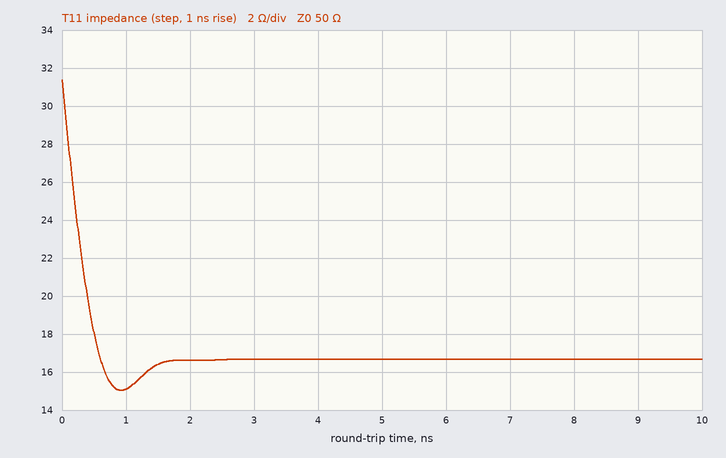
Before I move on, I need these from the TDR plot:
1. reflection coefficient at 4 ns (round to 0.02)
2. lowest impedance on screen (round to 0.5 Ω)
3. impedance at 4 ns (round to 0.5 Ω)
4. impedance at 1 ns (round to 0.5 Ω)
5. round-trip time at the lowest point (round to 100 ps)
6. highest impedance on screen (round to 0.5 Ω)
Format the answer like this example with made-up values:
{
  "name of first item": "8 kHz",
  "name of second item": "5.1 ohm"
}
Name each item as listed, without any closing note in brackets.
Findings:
{
  "reflection coefficient at 4 ns": "-0.50",
  "lowest impedance on screen": "15.0 Ω",
  "impedance at 4 ns": "16.5 Ω",
  "impedance at 1 ns": "15.0 Ω",
  "round-trip time at the lowest point": "900 ps",
  "highest impedance on screen": "31.5 Ω"
}
